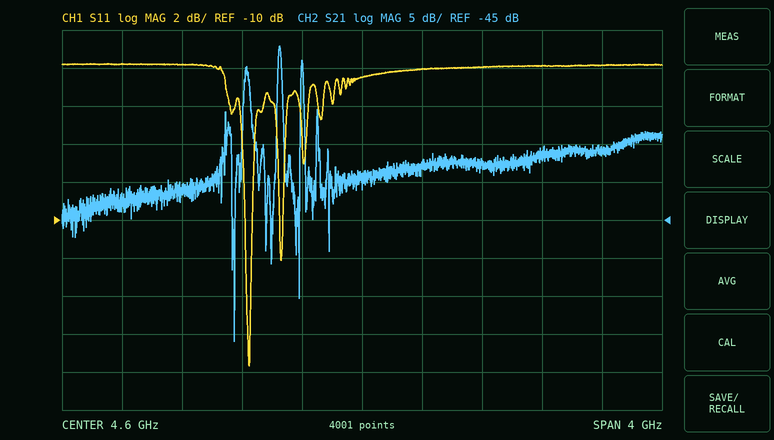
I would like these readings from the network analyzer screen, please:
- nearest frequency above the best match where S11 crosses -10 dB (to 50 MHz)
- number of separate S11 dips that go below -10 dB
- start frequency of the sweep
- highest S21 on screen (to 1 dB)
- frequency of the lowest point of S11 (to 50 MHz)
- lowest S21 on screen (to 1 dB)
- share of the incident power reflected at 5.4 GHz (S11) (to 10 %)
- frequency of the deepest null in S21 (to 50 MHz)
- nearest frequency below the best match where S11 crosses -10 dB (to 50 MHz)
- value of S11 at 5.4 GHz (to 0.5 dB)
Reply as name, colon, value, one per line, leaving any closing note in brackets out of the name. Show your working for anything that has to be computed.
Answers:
nearest frequency above the best match where S11 crosses -10 dB: 3.85 GHz
number of separate S11 dips that go below -10 dB: 2
start frequency of the sweep: 2.6 GHz
highest S21 on screen: -22 dB
frequency of the lowest point of S11: 3.85 GHz
lowest S21 on screen: -61 dB
share of the incident power reflected at 5.4 GHz (S11): 10^(-2/10) ≈ 63.1 %, so 60 % to the nearest 10 %
frequency of the deepest null in S21: 3.75 GHz
nearest frequency below the best match where S11 crosses -10 dB: 3.80 GHz
value of S11 at 5.4 GHz: -2.0 dB
